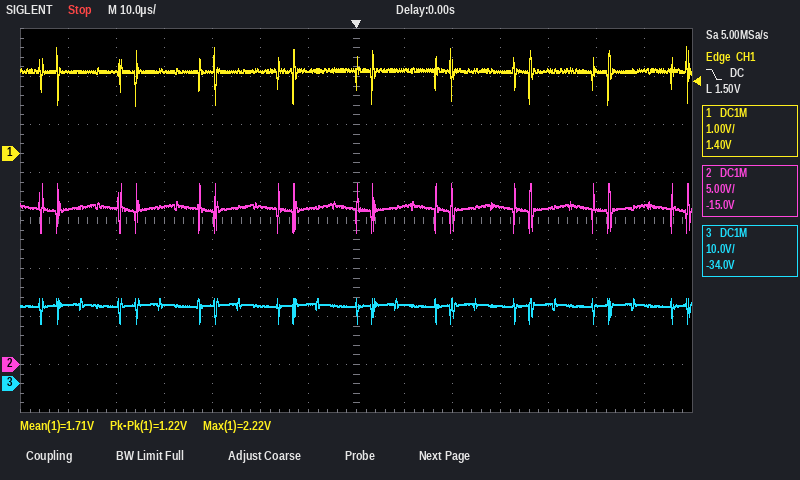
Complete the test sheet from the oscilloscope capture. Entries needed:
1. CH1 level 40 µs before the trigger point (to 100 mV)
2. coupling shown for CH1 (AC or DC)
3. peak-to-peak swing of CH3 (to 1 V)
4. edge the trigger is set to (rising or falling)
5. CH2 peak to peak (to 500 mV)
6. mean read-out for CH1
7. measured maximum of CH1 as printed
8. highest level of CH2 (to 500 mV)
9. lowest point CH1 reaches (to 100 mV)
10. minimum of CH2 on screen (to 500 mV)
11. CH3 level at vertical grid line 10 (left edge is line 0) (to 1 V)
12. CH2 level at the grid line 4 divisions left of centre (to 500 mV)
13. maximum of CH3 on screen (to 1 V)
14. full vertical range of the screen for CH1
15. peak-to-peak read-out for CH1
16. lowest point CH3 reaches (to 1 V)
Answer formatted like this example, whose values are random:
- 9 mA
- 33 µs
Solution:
- 1.7 V
- DC
- 5 V
- falling
- 5.0 V
- 1.71 V
- 2.22 V
- 19.0 V
- 1.0 V
- 14.0 V
- 16 V
- 16.5 V
- 18 V
- 8 V
- 1.22 V
- 13 V
